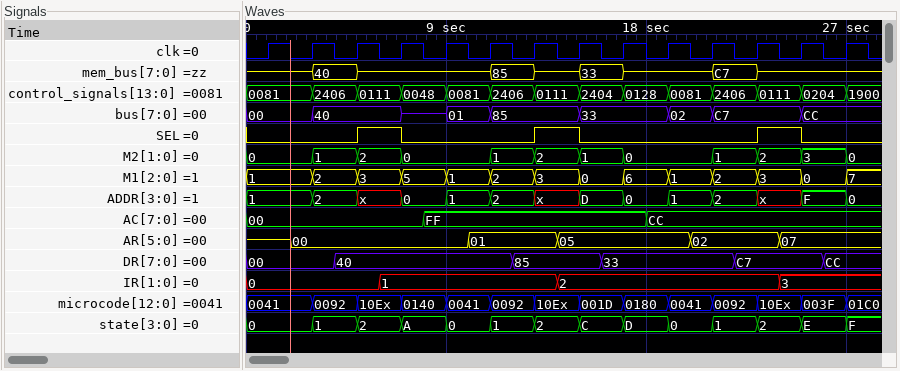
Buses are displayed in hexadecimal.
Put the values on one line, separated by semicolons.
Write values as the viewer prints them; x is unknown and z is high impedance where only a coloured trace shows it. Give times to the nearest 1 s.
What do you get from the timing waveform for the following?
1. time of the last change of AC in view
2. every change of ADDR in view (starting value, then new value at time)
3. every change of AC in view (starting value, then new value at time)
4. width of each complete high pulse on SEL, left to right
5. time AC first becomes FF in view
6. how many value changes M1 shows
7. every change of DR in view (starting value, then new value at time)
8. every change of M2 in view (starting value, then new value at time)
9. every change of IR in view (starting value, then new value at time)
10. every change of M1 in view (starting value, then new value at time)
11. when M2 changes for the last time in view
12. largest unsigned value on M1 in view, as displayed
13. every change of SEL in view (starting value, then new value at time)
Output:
18 s; 1, 2 at 3 s, x at 5 s, 0 at 7 s, 1 at 9 s, 2 at 11 s, x at 13 s, D at 15 s, 0 at 17 s, 1 at 19 s, 2 at 21 s, x at 23 s, F at 25 s, 0 at 27 s; 00, FF at 8 s, CC at 18 s; 2 s, 2 s, 2 s; 8 s; 13; 00, 40 at 4 s, 85 at 12 s, 33 at 16 s, C7 at 22 s, CC at 26 s; 0, 1 at 3 s, 2 at 5 s, 0 at 7 s, 1 at 11 s, 2 at 13 s, 1 at 15 s, 0 at 17 s, 1 at 21 s, 2 at 23 s, 3 at 25 s, 0 at 27 s; 0, 1 at 6 s, 2 at 14 s, 3 at 24 s; 1, 2 at 3 s, 3 at 5 s, 5 at 7 s, 1 at 9 s, 2 at 11 s, 3 at 13 s, 0 at 15 s, 6 at 17 s, 1 at 19 s, 2 at 21 s, 3 at 23 s, 0 at 25 s, 7 at 27 s; 27 s; 7; 0, 1 at 5 s, 0 at 7 s, 1 at 13 s, 0 at 15 s, 1 at 23 s, 0 at 25 s
